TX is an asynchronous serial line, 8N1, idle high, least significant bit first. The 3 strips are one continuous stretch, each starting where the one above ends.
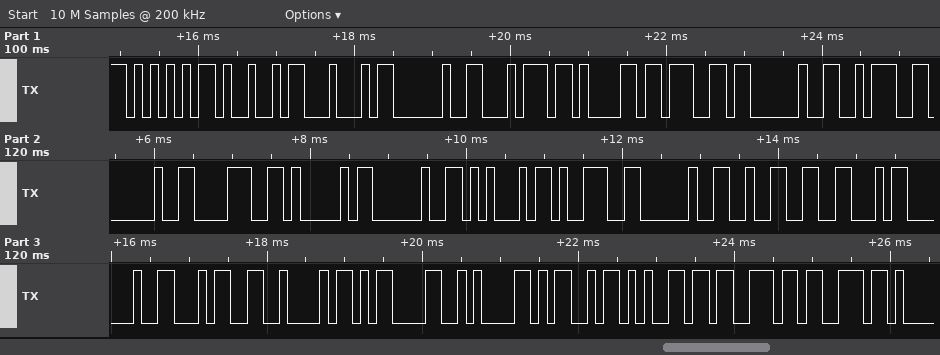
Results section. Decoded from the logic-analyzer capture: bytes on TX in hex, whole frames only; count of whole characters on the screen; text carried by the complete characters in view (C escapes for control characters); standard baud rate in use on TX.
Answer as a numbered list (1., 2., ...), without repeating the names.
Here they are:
1. 55 49 44 20 74 61 67 20 3A 20 38 41 20 45 39 20 32 46 20 34 42 0D 0A 4D 65 73 73
2. 27
3. "UID tag : 8A E9 2F 4B\r\nMess"
4. 9600 baud
